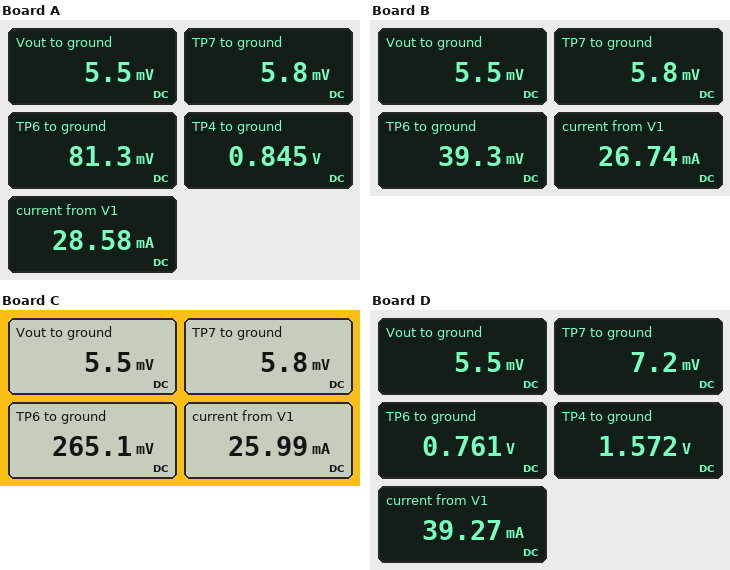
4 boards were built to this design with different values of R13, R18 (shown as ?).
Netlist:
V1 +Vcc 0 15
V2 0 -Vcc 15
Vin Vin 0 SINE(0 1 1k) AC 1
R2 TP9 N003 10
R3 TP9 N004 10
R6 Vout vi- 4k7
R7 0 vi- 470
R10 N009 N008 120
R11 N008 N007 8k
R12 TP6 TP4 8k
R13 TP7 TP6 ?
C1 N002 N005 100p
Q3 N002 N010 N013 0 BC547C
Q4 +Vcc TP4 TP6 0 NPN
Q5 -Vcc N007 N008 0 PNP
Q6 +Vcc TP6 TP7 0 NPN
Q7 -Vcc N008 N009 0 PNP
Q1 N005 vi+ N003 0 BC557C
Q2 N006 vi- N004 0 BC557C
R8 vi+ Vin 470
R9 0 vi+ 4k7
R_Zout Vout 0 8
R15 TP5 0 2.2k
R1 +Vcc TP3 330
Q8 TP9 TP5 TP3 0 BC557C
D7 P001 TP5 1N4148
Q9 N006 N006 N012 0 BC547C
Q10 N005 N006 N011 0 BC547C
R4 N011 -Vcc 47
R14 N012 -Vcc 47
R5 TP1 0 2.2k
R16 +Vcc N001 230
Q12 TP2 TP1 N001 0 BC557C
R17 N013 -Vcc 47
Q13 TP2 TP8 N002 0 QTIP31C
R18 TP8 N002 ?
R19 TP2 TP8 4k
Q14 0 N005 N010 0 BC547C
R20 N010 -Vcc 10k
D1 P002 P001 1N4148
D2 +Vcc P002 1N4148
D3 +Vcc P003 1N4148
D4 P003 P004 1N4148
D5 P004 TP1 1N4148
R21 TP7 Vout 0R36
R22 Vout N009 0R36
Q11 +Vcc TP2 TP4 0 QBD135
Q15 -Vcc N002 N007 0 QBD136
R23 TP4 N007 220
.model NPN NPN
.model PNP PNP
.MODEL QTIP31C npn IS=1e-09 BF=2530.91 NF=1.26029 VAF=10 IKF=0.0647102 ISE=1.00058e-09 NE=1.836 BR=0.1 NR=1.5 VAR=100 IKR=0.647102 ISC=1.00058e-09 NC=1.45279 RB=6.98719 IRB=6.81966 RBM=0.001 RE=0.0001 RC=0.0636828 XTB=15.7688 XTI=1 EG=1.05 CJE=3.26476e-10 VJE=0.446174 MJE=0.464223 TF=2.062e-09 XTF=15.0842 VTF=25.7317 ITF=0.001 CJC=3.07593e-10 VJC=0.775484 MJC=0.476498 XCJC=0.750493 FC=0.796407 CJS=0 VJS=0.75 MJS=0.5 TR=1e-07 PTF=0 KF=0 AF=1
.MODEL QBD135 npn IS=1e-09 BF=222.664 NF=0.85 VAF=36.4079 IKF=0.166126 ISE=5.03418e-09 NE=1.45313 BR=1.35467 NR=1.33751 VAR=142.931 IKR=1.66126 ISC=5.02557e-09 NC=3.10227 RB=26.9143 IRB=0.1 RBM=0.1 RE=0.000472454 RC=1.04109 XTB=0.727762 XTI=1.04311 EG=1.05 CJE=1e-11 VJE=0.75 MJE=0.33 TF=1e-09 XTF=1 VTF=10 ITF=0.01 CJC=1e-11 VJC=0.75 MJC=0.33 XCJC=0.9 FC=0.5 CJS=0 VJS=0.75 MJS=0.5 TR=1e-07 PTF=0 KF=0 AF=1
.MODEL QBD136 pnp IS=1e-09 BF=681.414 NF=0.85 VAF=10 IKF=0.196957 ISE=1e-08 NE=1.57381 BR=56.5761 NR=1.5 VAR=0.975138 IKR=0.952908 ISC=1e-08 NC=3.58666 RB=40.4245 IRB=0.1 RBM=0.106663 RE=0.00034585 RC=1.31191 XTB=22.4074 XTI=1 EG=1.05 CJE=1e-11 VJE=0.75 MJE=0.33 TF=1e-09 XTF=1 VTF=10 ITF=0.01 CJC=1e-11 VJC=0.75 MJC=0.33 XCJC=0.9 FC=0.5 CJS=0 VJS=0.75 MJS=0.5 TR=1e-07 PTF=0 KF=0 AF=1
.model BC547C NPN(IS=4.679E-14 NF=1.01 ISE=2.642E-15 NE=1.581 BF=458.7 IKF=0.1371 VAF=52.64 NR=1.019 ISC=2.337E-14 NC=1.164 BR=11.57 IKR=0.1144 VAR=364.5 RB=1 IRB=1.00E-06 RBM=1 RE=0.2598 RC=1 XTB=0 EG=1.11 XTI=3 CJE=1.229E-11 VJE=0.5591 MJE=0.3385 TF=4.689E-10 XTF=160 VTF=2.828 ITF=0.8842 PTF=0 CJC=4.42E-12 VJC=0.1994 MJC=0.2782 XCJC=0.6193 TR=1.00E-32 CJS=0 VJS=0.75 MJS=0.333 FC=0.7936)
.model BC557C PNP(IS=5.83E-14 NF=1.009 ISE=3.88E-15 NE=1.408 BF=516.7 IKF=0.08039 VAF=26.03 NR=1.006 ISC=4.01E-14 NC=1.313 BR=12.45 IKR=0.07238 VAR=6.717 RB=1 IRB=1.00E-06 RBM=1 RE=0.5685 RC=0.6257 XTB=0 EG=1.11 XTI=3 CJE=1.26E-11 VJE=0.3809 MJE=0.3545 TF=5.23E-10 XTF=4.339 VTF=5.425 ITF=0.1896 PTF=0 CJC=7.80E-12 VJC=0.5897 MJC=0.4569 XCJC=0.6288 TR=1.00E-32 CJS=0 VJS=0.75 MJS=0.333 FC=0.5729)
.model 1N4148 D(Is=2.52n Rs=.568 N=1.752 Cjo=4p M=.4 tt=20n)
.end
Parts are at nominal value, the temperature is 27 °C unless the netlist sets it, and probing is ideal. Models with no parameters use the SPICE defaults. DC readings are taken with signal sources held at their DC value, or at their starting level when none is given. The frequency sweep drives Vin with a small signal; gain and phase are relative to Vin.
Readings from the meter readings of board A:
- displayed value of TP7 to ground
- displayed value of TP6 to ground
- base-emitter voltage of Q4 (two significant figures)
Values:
5.8 mV
81.3 mV
760 mV
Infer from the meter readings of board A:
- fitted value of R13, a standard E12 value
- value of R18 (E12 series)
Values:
100 Ω
1.5 kΩ
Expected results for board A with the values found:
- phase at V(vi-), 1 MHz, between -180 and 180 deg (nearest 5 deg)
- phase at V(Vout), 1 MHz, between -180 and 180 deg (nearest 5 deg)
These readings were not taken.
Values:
-80 deg
-80 deg
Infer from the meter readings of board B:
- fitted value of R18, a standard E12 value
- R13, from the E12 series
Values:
2.2 kΩ
47 Ω
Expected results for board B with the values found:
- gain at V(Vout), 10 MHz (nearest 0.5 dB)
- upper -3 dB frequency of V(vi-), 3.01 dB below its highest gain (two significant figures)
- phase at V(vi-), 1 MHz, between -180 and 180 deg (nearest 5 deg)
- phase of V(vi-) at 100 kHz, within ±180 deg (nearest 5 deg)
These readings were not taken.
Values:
-9.5 dB
510 kHz
-70 deg
-10 deg
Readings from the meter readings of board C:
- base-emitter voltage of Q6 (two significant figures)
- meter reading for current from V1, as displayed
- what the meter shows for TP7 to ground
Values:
260 mV
25.99 mA
5.8 mV
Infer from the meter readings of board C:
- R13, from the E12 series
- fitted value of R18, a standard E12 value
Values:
390 Ω
2.7 kΩ
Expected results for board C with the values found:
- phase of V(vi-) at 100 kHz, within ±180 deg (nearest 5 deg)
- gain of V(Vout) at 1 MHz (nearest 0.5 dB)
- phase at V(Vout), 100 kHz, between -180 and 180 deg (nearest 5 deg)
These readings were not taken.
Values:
-40 deg
1.0 dB
-40 deg
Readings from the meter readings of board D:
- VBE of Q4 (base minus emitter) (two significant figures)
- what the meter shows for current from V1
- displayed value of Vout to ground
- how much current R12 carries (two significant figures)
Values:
810 mV
39.27 mA
5.5 mV
100 µA
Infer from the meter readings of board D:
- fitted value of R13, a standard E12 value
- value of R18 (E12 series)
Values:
180 Ω
680 Ω
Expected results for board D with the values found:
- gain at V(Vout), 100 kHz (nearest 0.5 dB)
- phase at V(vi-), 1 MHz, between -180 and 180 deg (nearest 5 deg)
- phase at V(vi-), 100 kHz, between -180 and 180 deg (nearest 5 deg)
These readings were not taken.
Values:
20.0 dB
-45 deg
-5 deg
